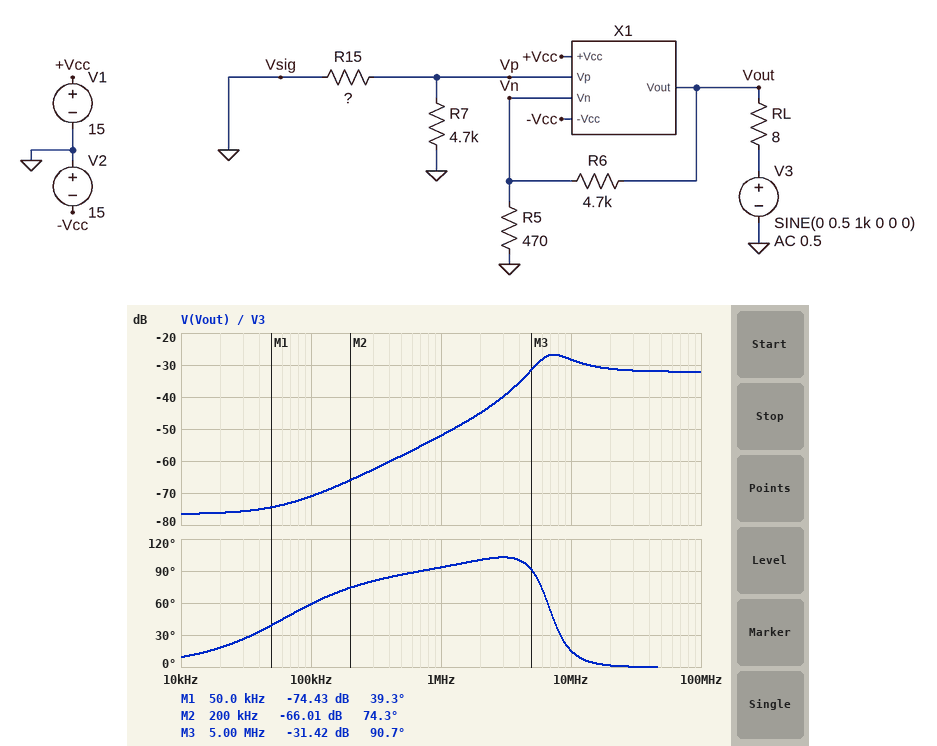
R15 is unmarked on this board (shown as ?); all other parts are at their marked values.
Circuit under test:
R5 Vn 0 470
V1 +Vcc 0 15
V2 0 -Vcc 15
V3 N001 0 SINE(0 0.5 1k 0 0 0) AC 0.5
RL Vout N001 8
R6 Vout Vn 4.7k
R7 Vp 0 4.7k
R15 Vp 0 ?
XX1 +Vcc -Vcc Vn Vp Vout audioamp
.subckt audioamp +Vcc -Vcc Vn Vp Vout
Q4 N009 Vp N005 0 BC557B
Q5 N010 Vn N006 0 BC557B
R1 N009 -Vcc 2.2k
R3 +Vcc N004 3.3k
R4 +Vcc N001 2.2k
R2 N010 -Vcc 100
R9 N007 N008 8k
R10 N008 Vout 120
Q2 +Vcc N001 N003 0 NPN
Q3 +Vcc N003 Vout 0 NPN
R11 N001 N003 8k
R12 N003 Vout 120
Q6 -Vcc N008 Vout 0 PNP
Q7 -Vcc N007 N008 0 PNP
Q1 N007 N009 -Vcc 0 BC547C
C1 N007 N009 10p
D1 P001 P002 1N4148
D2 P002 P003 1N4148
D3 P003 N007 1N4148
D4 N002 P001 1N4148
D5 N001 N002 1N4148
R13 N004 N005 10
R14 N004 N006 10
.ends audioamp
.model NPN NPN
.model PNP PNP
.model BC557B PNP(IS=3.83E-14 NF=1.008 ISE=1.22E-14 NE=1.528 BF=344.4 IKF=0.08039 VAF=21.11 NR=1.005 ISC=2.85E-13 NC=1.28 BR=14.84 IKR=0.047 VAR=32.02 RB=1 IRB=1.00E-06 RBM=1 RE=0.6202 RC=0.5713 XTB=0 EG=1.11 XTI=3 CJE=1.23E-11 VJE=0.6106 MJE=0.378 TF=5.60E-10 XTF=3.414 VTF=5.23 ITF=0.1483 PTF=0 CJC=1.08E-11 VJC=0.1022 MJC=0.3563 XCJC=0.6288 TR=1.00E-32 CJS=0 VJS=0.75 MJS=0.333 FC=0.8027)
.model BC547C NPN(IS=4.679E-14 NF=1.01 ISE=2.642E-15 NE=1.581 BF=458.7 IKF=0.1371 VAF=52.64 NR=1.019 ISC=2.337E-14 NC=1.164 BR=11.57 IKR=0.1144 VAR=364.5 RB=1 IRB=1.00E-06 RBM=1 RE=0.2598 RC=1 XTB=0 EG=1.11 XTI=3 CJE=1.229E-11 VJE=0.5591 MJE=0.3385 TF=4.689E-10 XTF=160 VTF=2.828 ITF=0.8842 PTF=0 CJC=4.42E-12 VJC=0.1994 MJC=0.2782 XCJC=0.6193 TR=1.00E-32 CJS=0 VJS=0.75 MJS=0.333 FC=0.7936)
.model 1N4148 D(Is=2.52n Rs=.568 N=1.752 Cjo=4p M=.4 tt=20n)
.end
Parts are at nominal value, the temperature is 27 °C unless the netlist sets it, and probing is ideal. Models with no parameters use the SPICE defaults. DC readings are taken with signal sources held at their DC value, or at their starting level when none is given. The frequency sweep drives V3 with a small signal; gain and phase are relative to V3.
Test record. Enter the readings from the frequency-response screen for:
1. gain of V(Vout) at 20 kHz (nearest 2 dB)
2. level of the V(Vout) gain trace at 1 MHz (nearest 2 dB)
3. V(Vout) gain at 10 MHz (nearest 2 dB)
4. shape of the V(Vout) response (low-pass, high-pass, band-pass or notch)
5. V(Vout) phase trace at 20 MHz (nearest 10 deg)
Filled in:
-76 dB
-52 dB
-28 dB
high-pass
0 deg
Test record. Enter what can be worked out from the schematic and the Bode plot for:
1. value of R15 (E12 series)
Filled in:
1.5 kΩ
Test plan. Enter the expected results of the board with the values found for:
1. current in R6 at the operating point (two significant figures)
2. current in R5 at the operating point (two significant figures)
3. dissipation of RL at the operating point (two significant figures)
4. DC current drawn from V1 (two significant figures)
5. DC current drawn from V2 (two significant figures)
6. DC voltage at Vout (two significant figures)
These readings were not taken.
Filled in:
230 µA
230 µA
180 mW
21 mA
170 mA
-1.2 V
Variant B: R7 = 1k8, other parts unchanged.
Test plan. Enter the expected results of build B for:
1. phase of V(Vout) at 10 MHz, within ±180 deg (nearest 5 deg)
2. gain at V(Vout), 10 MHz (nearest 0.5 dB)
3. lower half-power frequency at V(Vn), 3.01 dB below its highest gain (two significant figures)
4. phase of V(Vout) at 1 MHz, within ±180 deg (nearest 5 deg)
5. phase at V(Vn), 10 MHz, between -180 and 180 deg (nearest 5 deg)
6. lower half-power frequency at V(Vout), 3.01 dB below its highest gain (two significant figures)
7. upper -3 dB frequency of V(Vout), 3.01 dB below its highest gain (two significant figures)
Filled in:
25 deg
-27.5 dB
6.1 MHz
90 deg
15 deg
6.2 MHz
16 MHz
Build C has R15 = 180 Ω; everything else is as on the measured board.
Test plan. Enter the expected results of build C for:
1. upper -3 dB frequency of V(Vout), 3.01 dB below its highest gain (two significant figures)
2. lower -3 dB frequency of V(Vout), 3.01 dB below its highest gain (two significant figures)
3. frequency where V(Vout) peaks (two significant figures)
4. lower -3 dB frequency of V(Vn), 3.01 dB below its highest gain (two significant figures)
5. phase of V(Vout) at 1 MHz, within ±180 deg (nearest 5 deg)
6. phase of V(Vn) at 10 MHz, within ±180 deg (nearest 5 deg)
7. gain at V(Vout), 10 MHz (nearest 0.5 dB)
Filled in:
58 MHz
9.2 MHz
16 MHz
8.5 MHz
85 deg
45 deg
-31.0 dB
